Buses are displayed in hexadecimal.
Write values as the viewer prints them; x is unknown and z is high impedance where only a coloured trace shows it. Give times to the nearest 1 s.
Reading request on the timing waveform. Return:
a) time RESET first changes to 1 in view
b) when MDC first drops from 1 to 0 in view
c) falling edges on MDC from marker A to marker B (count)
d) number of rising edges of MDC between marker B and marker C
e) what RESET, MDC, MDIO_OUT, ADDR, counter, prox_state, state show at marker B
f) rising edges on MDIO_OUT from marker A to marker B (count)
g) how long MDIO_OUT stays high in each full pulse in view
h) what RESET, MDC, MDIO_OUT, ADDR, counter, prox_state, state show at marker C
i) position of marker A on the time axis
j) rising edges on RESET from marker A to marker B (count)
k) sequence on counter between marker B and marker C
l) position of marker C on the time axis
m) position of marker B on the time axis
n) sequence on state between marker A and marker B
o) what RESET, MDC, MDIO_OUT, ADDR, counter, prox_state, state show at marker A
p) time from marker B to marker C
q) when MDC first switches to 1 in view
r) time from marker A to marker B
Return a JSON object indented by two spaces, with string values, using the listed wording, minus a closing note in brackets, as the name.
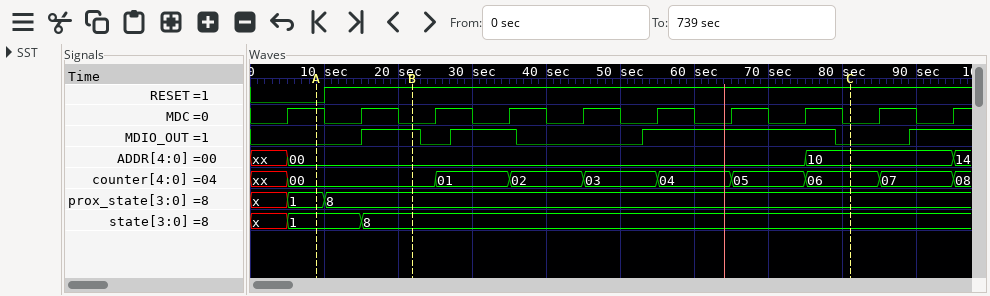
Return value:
{
  "time RESET first changes to 1 in view": "10 s",
  "when MDC first drops from 1 to 0 in view": "10 s",
  "falling edges on MDC from marker A to marker B": "2",
  "number of rising edges of MDC between marker B and marker C": "6",
  "what RESET, MDC, MDIO_OUT, ADDR, counter, prox_state, state show at marker B": "RESET=1, MDC=0, MDIO_OUT=1, ADDR=00, counter=00, prox_state=8, state=8",
  "rising edges on MDIO_OUT from marker A to marker B": "1",
  "how long MDIO_OUT stays high in each full pulse in view": "8 s, 9 s, 26 s",
  "what RESET, MDC, MDIO_OUT, ADDR, counter, prox_state, state show at marker C": "RESET=1, MDC=0, MDIO_OUT=0, ADDR=10, counter=06, prox_state=8, state=8",
  "position of marker A on the time axis": "9 s",
  "rising edges on RESET from marker A to marker B": "1",
  "sequence on counter between marker B and marker C": "00, 01, 02, 03, 04, 05, 06",
  "position of marker C on the time axis": "81 s",
  "position of marker B on the time axis": "22 s",
  "sequence on state between marker A and marker B": "1, 8",
  "what RESET, MDC, MDIO_OUT, ADDR, counter, prox_state, state show at marker A": "RESET=0, MDC=1, MDIO_OUT=0, ADDR=00, counter=00, prox_state=1, state=1",
  "time from marker B to marker C": "59 s",
  "when MDC first switches to 1 in view": "5 s",
  "time from marker A to marker B": "13 s"
}
